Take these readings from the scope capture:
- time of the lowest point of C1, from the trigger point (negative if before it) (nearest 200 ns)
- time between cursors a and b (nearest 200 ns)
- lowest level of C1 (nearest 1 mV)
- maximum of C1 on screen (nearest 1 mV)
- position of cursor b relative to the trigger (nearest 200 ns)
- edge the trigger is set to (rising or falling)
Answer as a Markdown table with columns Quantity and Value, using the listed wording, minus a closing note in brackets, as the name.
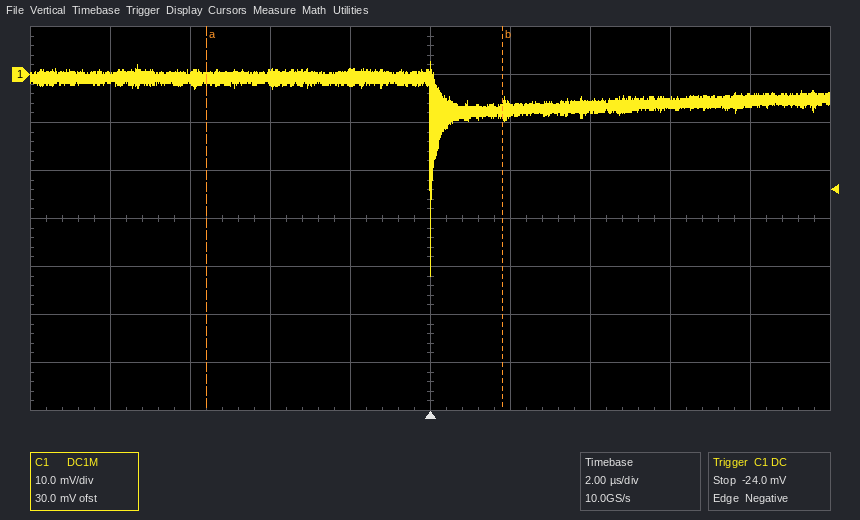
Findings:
| Quantity | Value |
|---|---|
| time of the lowest point of C1, from the trigger point (negative if before it) | 0.0 µs |
| time between cursors a and b | 7.4 µs |
| lowest level of C1 | -42 mV |
| maximum of C1 on screen | 3 mV |
| position of cursor b relative to the trigger | +1.8 µs |
| edge the trigger is set to | falling |
